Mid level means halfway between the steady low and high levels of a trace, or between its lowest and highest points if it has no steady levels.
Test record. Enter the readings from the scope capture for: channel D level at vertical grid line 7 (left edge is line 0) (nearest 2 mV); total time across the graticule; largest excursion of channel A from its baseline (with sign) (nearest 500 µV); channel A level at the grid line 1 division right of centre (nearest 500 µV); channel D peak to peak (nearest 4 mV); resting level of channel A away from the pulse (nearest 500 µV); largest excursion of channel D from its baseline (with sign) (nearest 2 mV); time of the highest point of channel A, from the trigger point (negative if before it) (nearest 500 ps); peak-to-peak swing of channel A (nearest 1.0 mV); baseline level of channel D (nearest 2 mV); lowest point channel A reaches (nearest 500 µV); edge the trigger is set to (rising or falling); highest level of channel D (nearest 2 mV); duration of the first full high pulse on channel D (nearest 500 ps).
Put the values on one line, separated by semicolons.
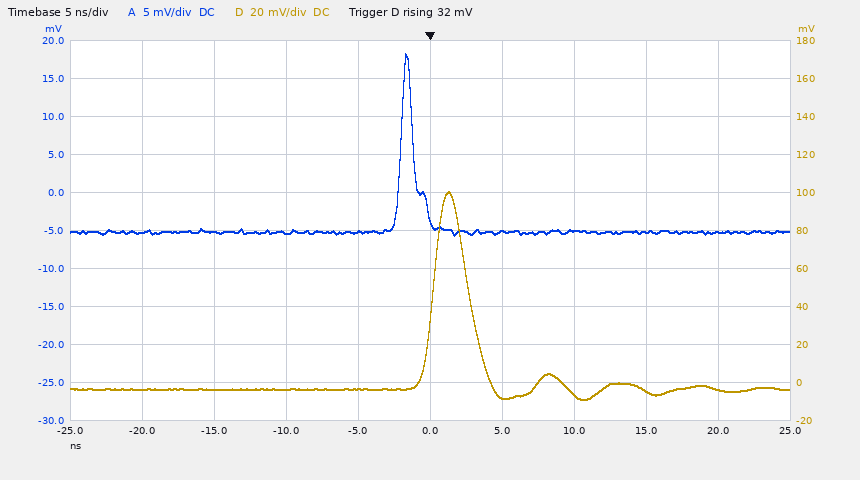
-6 mV; 50 ns; +23.5 mV; -5.0 mV; 108 mV; -5.0 mV; +104 mV; -1.5 ns; 24.0 mV; -4 mV; -5.5 mV; rising; 100 mV; 2.5 ns
